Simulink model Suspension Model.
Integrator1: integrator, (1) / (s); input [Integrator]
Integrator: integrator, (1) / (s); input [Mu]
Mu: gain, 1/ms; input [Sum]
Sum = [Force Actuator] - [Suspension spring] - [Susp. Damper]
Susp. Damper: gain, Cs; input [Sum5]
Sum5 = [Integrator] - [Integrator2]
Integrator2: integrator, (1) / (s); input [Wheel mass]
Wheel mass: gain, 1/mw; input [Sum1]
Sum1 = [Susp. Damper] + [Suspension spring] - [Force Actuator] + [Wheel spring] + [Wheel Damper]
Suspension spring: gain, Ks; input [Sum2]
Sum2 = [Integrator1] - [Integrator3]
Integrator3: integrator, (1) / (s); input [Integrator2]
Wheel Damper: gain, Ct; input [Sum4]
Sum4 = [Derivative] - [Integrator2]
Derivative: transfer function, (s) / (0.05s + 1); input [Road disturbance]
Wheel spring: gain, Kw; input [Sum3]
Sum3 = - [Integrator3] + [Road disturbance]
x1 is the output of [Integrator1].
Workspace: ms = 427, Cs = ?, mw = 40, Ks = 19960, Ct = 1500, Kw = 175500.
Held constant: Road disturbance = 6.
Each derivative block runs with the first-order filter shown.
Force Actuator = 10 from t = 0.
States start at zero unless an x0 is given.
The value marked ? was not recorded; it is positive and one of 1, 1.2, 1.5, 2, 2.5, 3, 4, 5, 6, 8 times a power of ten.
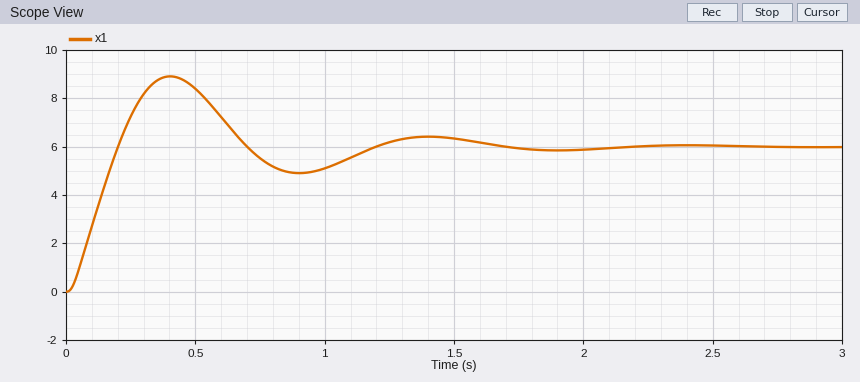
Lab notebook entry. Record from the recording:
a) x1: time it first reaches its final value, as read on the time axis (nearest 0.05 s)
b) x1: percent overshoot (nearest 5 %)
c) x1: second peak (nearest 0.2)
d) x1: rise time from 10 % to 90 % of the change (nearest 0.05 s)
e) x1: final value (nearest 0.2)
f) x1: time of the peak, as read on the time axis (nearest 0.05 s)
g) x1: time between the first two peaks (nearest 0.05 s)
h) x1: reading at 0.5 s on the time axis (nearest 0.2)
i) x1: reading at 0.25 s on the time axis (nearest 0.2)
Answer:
0.20 s
50 %
6.4
0.15 s
6.0
0.40 s
1.00 s
8.4
7.2
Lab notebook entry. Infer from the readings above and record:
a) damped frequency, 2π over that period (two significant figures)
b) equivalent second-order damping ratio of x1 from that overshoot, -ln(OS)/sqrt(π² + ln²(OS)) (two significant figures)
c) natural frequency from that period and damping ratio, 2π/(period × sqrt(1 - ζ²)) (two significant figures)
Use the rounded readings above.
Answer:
6.3 rad/s
0.22
6.4 rad/s
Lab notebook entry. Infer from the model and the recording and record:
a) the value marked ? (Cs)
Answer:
2000
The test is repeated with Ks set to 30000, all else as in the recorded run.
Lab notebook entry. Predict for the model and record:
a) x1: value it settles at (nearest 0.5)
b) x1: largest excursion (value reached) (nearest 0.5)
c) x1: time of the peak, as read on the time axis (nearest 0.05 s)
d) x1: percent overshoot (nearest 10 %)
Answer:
6.0
9.5
0.35 s
60 %
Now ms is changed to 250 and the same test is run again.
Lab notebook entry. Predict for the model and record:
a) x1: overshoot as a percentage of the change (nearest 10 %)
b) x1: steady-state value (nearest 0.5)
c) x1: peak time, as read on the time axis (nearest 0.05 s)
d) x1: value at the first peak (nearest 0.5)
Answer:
40 %
6.0
0.30 s
8.5
